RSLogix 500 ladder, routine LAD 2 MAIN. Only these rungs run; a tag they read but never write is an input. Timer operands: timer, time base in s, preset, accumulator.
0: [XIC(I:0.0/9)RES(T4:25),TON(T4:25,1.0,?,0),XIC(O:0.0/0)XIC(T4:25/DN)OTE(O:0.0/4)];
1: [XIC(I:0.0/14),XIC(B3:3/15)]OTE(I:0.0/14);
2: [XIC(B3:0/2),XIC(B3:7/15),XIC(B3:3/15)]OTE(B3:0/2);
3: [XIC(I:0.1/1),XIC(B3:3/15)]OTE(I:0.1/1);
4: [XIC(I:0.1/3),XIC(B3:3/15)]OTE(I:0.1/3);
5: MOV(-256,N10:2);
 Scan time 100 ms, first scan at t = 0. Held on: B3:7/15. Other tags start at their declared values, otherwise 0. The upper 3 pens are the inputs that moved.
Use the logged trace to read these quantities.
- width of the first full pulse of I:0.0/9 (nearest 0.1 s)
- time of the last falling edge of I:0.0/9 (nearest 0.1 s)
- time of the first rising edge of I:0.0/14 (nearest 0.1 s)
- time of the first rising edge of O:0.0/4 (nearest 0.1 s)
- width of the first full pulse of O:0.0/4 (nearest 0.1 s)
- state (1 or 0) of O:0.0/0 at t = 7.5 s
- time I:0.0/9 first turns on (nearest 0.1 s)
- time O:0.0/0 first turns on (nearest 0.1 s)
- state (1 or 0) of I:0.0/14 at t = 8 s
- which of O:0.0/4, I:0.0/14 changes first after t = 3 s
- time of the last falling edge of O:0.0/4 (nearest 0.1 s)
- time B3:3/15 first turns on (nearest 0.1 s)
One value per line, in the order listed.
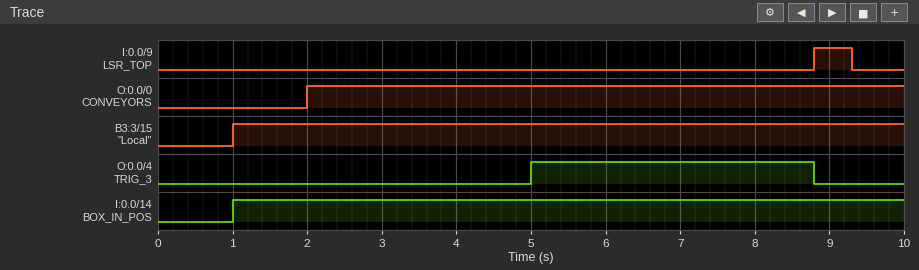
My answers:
0.5 s
9.3 s
1.0 s
5.0 s
3.8 s
1
8.8 s
2.0 s
1
O:0.0/4
8.8 s
1.0 s
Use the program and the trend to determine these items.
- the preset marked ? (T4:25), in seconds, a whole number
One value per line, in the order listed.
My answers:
5 s
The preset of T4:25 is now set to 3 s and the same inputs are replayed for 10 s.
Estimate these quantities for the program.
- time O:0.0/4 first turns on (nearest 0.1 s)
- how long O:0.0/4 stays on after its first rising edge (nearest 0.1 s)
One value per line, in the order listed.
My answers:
3.0 s
5.8 s
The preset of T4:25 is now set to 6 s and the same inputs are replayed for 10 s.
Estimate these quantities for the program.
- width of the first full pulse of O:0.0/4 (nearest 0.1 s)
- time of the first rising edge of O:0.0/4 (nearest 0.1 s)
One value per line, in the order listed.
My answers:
2.8 s
6.0 s
